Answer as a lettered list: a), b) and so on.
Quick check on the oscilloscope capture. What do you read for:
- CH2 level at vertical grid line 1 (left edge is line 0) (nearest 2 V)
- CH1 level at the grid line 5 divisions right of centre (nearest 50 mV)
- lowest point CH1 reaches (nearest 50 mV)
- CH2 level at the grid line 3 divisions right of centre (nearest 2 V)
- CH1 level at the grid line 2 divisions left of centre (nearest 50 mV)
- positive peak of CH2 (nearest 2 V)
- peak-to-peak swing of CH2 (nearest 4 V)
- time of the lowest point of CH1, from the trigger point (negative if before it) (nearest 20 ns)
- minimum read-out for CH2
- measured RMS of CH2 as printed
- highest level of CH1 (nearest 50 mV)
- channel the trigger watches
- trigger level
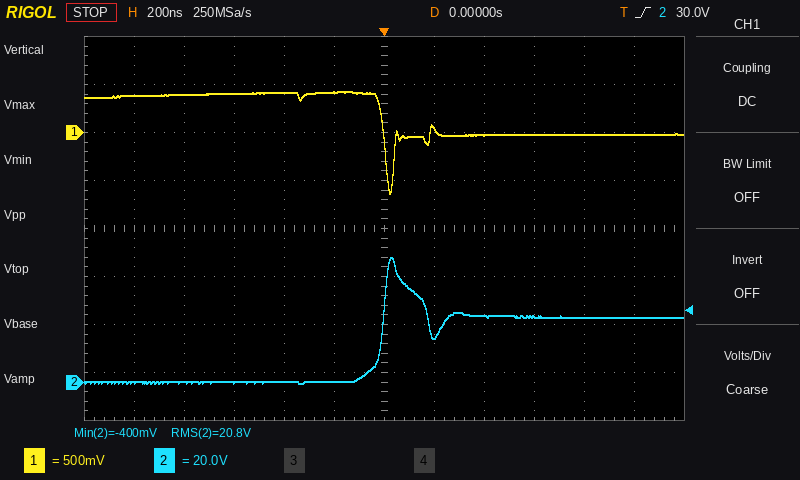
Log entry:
a) 0 V
b) 0 mV
c) -650 mV
d) 28 V
e) 400 mV
f) 52 V
g) 52 V
h) +20 ns
i) -400 mV
j) 20.8 V
k) 450 mV
l) CH2
m) 30.0 V
